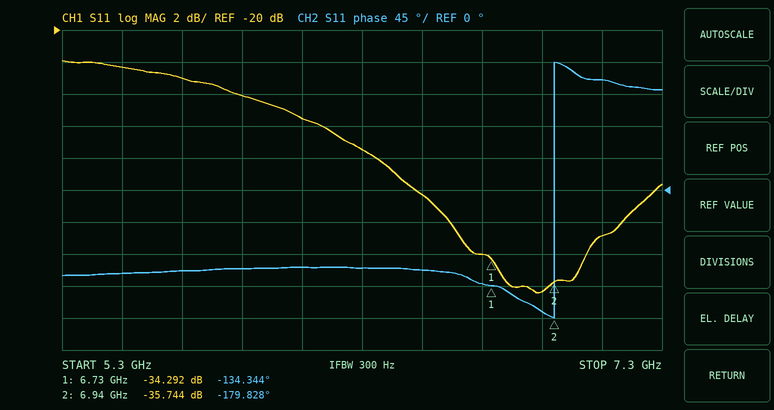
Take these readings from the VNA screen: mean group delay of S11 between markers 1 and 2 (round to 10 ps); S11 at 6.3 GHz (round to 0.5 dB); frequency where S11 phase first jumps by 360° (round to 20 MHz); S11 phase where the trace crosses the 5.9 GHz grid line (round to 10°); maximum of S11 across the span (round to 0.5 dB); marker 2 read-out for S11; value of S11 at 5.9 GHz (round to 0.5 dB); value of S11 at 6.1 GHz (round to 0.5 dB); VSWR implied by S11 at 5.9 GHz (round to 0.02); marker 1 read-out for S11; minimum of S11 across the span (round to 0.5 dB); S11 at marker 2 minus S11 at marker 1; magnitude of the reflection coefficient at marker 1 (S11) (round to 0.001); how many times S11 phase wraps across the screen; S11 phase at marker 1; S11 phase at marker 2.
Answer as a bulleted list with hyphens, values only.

- 600 ps
- -27.5 dB
- 6.94 GHz
- -110°
- -22.0 dB
- -35.744 dB
- -24.0 dB
- -25.5 dB
- 1.14
- -34.292 dB
- -36.5 dB
- -1.452 dB
- 0.019
- 1
- -134.344°
- -179.828°
